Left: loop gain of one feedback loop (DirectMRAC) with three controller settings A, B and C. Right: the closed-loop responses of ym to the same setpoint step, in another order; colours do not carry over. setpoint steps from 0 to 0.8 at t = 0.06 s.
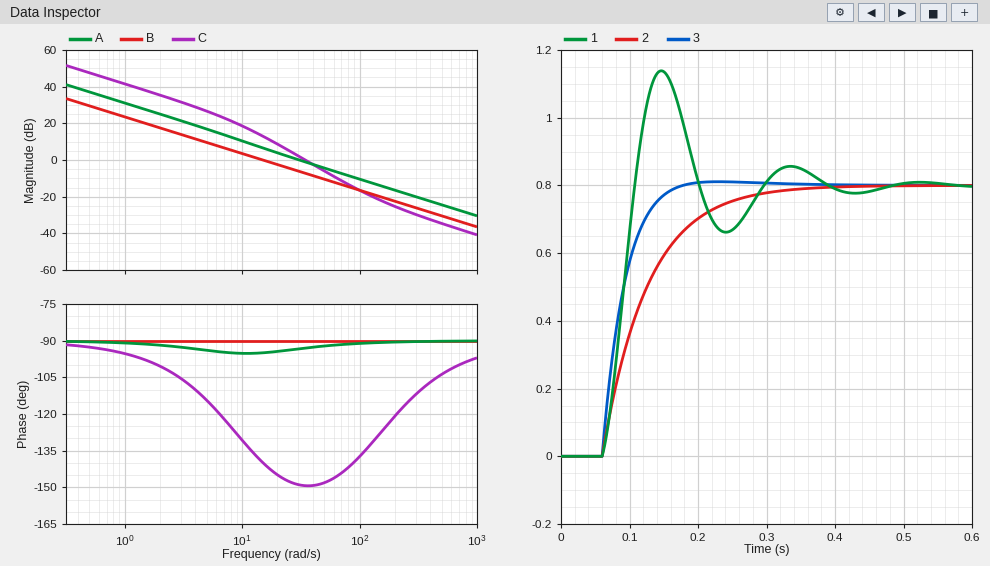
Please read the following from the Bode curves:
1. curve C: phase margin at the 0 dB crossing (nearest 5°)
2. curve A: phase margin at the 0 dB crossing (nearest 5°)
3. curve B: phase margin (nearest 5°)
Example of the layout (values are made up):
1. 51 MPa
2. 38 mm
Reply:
1. 30°
2. 85°
3. 90°
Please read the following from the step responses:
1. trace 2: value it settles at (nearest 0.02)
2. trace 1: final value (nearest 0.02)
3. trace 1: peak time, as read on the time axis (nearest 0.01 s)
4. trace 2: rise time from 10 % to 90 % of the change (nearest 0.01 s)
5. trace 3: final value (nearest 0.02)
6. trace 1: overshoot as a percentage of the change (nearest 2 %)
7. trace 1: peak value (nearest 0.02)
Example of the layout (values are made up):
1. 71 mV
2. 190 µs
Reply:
1. 0.80
2. 0.80
3. 0.15 s
4. 0.15 s
5. 0.80
6. 42 %
7. 1.14
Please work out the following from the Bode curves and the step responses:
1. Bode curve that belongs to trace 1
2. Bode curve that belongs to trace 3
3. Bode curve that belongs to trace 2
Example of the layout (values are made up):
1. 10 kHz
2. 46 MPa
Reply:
1. C
2. A
3. B
